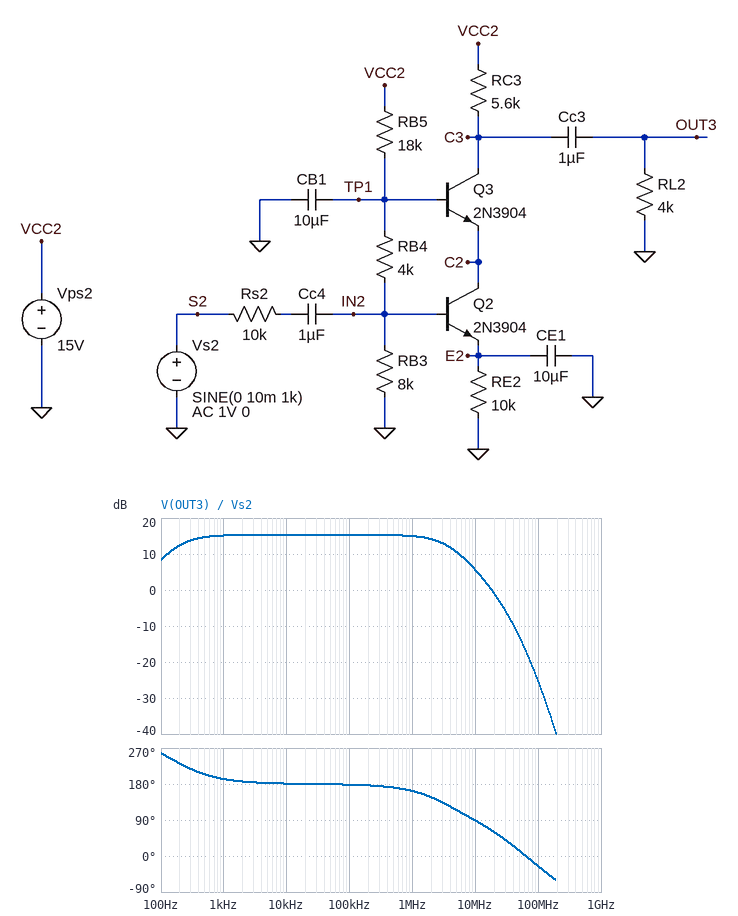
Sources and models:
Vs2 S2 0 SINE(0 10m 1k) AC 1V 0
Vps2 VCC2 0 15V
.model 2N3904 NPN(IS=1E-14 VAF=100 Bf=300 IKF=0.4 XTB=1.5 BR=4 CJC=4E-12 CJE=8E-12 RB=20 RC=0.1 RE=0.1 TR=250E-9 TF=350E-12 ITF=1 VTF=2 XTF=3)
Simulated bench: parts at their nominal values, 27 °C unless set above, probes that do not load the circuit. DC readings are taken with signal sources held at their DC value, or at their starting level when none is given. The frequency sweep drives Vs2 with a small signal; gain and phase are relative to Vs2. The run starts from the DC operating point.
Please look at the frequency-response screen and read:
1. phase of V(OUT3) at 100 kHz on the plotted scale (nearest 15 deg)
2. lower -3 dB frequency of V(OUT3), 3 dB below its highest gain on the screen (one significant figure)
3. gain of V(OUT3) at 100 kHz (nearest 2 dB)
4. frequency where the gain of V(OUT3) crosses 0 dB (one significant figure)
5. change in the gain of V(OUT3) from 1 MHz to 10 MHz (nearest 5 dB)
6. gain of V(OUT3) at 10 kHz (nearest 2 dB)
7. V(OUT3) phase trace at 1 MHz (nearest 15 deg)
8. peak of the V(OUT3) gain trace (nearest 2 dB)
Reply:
180 deg
200 Hz
16 dB
20 MHz
-10 dB
16 dB
165 deg
16 dB
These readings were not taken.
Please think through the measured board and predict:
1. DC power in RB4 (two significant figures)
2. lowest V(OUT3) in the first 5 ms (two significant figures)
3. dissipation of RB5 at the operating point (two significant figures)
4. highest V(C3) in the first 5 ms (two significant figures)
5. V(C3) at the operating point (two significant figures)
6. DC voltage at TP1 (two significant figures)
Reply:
1.0 mW
-58 mV
4.5 mW
13 V
13 V
6.0 V
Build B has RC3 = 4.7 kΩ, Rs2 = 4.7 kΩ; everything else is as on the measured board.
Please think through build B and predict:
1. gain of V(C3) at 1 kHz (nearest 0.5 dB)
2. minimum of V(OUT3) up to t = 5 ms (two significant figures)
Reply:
19.5 dB
-95 mV
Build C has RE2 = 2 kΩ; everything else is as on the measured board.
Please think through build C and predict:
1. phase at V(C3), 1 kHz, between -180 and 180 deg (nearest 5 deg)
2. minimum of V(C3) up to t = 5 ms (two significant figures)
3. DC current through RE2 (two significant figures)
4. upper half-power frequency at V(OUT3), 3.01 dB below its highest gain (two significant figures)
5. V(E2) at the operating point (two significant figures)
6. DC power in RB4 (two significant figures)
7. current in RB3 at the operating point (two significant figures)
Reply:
-145 deg
5.7 V
1.6 mA
2.6 MHz
3.3 V
990 µW
490 µA
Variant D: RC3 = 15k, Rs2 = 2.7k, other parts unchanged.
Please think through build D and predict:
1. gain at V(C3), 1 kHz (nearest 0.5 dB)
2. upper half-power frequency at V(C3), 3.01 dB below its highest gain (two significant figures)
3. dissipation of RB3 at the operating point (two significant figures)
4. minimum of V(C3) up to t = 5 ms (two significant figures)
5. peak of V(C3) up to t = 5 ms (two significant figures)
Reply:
25.5 dB
5.2 MHz
2.0 mW
9.8 V
10 V
